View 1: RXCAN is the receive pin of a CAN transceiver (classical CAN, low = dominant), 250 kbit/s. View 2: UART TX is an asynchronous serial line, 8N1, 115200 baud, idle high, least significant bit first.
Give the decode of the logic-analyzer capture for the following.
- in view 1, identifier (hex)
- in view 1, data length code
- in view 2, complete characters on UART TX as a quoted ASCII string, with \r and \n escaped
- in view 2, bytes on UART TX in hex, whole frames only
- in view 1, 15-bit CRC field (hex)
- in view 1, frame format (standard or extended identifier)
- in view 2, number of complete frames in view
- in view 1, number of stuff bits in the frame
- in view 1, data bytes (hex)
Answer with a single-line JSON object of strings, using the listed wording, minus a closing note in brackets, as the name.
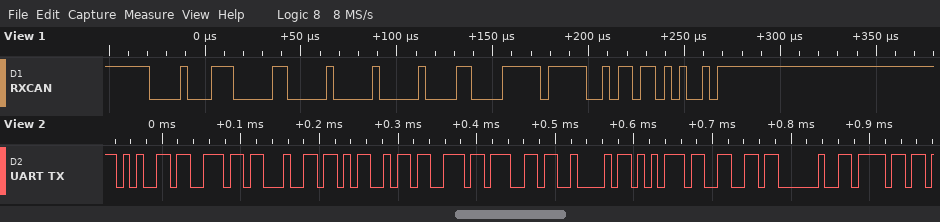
{"in view 1, identifier": "0x08E", "in view 1, data length code": "4", "in view 2, complete characters on UART TX as a quoted ASCII string, with \\r and \\n escaped": "\"endMsgBuf o\"", "in view 2, bytes on UART TX in hex, whole frames only": "65 6E 64 4D 73 67 42 75 66 20 6F", "in view 1, 15-bit CRC field": "0x56D4", "in view 1, frame format": "standard", "in view 2, number of complete frames in view": "11", "in view 1, number of stuff bits in the frame": "6", "in view 1, data bytes": "00 00 61 FF"}
